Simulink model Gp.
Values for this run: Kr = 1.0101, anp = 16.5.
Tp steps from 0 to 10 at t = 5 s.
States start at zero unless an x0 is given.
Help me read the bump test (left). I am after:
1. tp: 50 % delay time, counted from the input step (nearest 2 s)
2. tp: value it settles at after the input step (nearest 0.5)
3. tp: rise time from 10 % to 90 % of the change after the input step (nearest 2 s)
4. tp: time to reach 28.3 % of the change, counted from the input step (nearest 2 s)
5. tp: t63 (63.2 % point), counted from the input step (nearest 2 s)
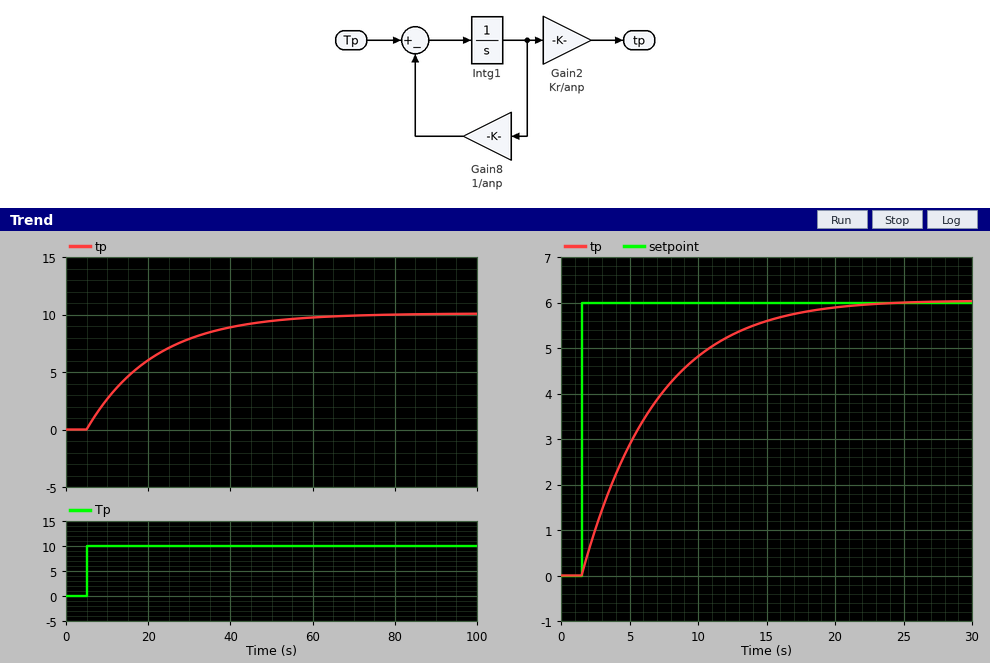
12 s
10.0
36 s
6 s
16 s
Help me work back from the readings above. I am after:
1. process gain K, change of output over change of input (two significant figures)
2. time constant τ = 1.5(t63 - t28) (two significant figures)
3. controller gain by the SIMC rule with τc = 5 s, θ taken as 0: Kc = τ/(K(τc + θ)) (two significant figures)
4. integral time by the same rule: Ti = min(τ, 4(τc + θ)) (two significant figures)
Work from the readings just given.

1.0
15 s
3.0
15 s
